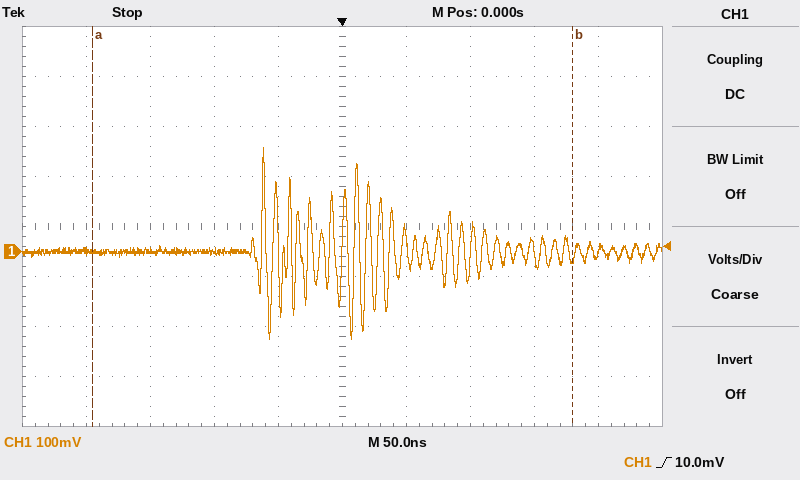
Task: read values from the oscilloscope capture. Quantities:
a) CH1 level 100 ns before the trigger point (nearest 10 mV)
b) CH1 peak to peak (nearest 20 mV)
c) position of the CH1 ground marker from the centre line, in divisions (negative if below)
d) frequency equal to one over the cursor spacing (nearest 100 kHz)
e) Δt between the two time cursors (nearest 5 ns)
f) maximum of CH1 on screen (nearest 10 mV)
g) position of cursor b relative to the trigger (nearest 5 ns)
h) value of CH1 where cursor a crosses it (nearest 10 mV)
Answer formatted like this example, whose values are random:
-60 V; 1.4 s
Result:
0 mV; 380 mV; -0.5 div; 2.7 MHz; 375 ns; 210 mV; +180 ns; 0 mV
